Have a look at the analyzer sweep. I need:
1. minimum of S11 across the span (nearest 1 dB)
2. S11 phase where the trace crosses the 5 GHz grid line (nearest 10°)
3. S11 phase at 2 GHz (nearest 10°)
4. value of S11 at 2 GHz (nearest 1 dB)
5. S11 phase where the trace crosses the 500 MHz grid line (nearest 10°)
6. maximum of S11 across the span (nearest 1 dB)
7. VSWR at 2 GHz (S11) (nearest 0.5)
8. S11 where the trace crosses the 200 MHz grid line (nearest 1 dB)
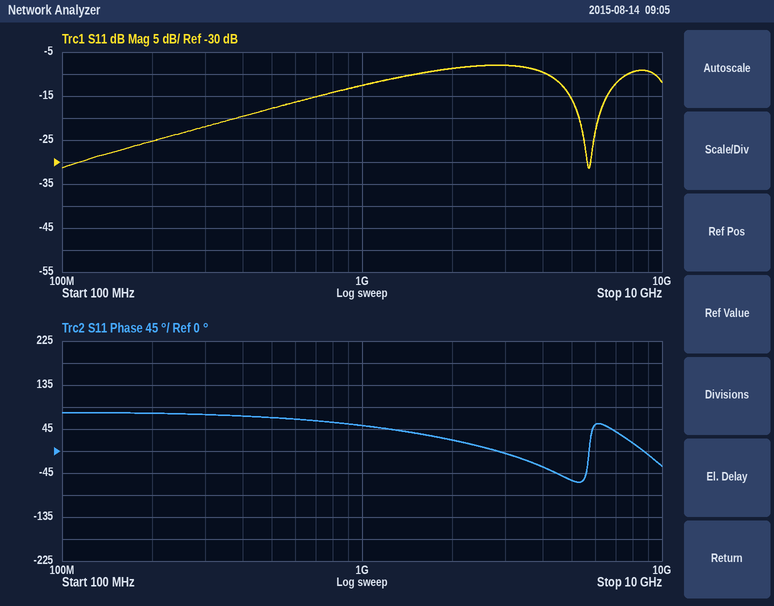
-31 dB
-60°
20°
-9 dB
70°
-8 dB
2.0
-25 dB
